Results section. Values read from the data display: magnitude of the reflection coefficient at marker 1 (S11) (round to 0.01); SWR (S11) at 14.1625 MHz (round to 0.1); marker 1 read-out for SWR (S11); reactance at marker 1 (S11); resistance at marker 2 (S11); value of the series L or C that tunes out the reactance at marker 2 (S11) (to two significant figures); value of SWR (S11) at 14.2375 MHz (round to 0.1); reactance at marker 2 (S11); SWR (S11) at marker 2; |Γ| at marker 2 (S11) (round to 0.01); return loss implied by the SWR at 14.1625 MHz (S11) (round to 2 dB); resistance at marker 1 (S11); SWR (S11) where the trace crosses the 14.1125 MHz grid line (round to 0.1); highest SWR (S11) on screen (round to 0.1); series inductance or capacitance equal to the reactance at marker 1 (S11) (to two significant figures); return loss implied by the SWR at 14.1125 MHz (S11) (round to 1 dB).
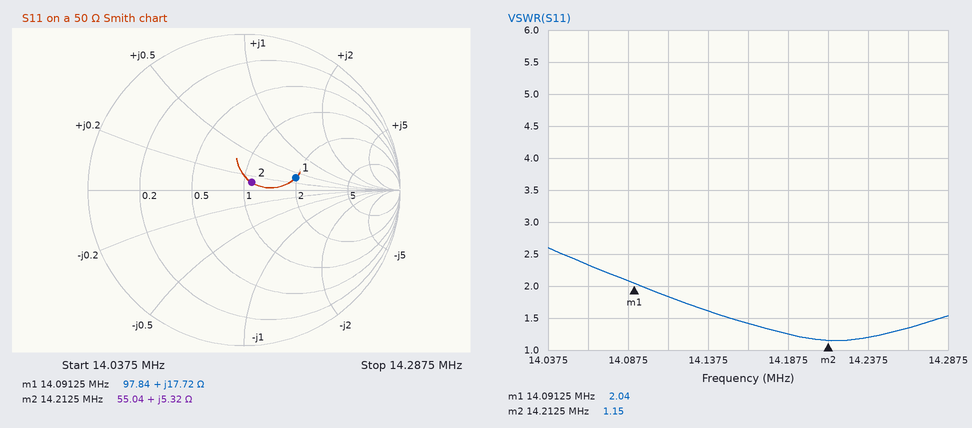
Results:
0.34
1.4
2.04
+17.72 Ω
55.04 Ω
2.1 nF
1.2
+5.32 Ω
1.15
0.07
16 dB
97.84 Ω
1.8
2.6
200 nH
11 dB
